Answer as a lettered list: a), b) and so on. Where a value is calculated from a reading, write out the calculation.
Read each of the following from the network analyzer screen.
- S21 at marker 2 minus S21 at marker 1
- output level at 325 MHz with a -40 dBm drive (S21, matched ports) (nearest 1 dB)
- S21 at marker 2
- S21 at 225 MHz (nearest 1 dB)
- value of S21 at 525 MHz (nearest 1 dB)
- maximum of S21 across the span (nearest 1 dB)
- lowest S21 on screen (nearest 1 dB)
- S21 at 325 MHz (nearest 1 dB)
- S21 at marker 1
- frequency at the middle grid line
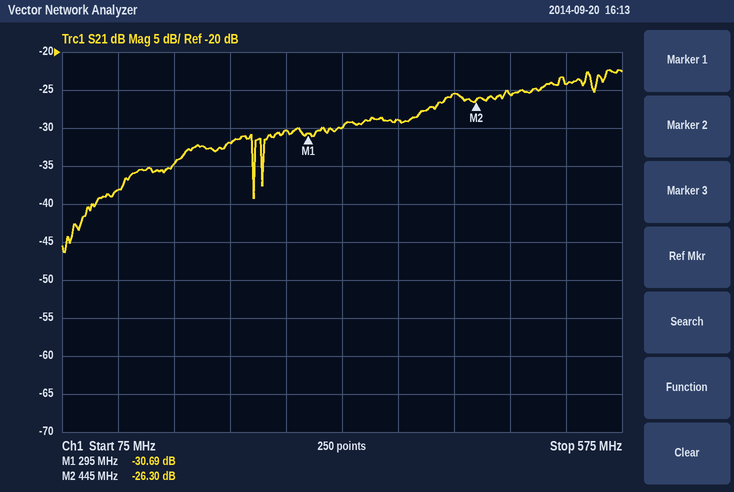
a) -26.3 − (-30.69) = 4.39 dB
b) -40 dBm + (-30 dB) = -70 dBm
c) -26.30 dB
d) -32 dB
e) -24 dB
f) -22 dB
g) -46 dB
h) -30 dB
i) -30.69 dB
j) 325 MHz
